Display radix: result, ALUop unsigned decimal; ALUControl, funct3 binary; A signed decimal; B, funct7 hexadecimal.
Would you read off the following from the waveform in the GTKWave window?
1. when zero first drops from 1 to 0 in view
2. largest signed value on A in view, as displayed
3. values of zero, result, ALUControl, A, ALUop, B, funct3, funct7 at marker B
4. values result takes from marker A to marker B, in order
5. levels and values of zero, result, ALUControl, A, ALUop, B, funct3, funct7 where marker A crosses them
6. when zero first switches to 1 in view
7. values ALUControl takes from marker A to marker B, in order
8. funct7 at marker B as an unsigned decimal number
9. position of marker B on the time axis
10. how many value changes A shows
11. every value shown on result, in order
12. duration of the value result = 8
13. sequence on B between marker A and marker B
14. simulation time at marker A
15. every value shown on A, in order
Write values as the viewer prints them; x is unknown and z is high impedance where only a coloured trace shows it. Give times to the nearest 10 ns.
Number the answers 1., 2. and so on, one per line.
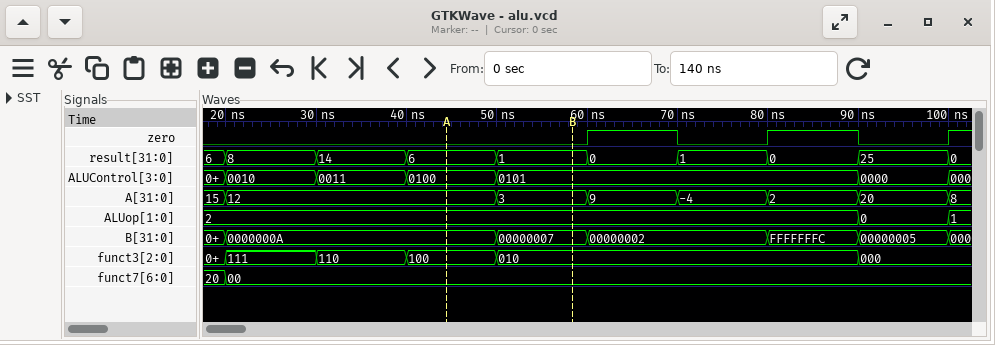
1. 70 ns
2. 20
3. zero=0, result=1, ALUControl=0101, A=3, ALUop=2, B=00000007, funct3=010, funct7=00
4. 6, 1
5. zero=0, result=6, ALUControl=0100, A=12, ALUop=2, B=0000000A, funct3=100, funct7=00
6. 60 ns
7. 0100, 0101
8. 0
9. 60 ns
10. 7
11. 6, 8, 14, 6, 1, 0, 1, 0, 25, 0
12. 10 ns
13. 0000000A, 00000007
14. 40 ns
15. 15, 12, 3, 9, -4, 2, 20, 8
